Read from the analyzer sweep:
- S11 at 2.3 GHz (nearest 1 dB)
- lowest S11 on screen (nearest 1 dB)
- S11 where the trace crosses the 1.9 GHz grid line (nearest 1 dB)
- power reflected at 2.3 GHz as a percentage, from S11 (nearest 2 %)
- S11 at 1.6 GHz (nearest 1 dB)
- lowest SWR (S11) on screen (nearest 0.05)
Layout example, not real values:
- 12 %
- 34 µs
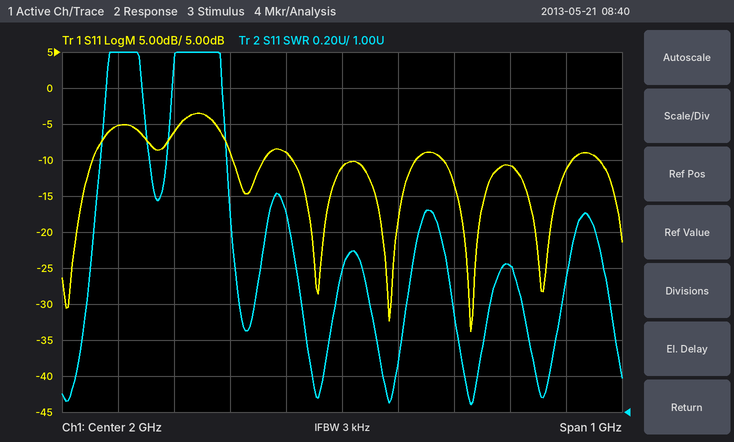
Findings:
- -11 dB
- -34 dB
- -9 dB
- 8 %
- -5 dB
- 1.05
